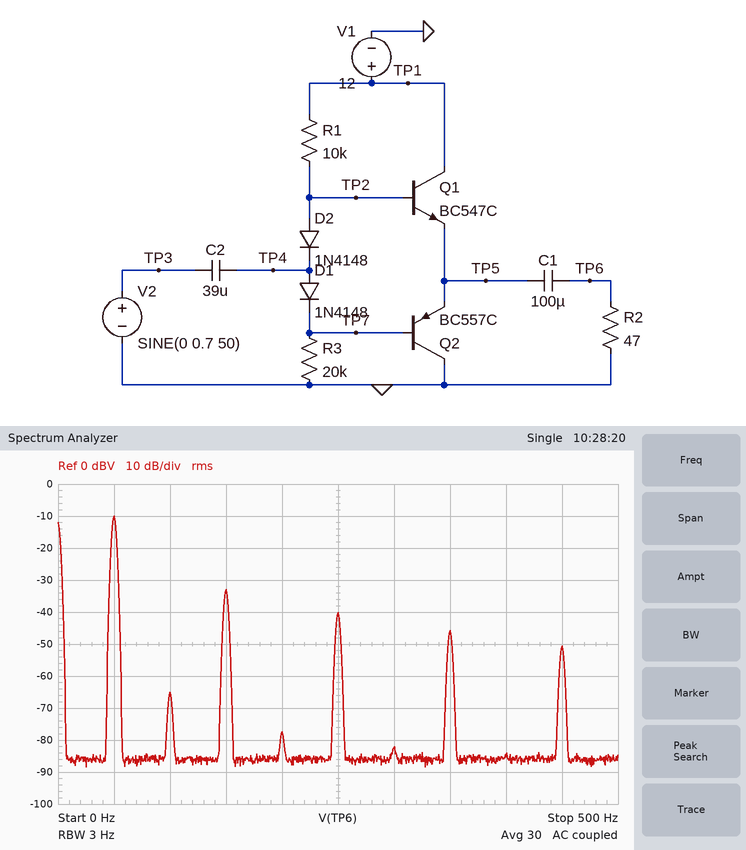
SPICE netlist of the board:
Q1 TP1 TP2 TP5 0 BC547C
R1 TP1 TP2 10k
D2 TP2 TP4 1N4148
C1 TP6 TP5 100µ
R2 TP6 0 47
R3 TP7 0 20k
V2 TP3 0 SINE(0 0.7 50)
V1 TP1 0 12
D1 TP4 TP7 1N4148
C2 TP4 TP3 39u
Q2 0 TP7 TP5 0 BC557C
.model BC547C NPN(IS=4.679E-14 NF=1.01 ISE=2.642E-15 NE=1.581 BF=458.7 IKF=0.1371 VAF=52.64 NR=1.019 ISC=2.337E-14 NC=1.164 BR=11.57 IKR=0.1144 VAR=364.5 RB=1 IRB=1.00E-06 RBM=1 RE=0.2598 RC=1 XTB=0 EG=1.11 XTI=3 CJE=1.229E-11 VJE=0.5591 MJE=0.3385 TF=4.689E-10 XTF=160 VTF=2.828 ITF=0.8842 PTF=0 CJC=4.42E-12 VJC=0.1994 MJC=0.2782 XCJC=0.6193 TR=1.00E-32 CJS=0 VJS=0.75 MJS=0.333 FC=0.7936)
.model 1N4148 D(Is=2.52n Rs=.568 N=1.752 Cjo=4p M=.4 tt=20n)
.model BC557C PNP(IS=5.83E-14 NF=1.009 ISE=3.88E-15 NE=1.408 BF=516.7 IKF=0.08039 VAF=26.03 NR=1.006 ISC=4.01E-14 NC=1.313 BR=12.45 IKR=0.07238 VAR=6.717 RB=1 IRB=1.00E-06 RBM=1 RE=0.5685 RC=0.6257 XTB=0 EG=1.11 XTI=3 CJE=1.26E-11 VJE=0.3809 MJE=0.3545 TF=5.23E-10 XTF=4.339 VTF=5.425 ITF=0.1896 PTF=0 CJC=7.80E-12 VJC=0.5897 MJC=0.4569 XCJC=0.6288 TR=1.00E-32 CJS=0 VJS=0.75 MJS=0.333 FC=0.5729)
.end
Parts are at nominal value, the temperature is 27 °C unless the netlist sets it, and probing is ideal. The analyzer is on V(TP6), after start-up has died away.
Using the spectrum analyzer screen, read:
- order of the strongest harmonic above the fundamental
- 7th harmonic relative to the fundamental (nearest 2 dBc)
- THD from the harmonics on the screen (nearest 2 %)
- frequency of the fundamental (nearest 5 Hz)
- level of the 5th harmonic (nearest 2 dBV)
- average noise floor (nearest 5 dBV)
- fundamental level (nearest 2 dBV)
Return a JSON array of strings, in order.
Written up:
["3", "-36 dBc", "8 %", "50 Hz", "-40 dBV", "-85 dBV", "-10 dBV"]
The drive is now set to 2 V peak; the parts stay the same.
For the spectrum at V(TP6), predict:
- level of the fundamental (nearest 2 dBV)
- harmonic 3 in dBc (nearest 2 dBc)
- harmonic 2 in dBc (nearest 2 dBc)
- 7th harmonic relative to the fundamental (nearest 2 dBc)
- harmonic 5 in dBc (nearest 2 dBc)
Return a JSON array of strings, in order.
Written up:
["0 dBV", "-30 dBc", "-48 dBc", "-40 dBc", "-36 dBc"]
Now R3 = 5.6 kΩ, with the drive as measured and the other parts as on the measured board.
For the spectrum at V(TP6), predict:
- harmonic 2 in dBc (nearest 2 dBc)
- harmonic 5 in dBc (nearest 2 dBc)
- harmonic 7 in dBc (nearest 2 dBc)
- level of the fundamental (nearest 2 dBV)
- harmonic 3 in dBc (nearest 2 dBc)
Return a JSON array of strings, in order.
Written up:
["-50 dBc", "-34 dBc", "-40 dBc", "-10 dBV", "-26 dBc"]
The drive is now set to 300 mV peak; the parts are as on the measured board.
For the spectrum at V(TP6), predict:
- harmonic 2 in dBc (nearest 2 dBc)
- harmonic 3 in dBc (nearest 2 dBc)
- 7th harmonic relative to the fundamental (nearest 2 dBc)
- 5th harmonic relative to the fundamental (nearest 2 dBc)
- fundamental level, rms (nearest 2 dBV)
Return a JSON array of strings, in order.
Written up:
["-58 dBc", "-18 dBc", "-38 dBc", "-28 dBc", "-20 dBV"]
